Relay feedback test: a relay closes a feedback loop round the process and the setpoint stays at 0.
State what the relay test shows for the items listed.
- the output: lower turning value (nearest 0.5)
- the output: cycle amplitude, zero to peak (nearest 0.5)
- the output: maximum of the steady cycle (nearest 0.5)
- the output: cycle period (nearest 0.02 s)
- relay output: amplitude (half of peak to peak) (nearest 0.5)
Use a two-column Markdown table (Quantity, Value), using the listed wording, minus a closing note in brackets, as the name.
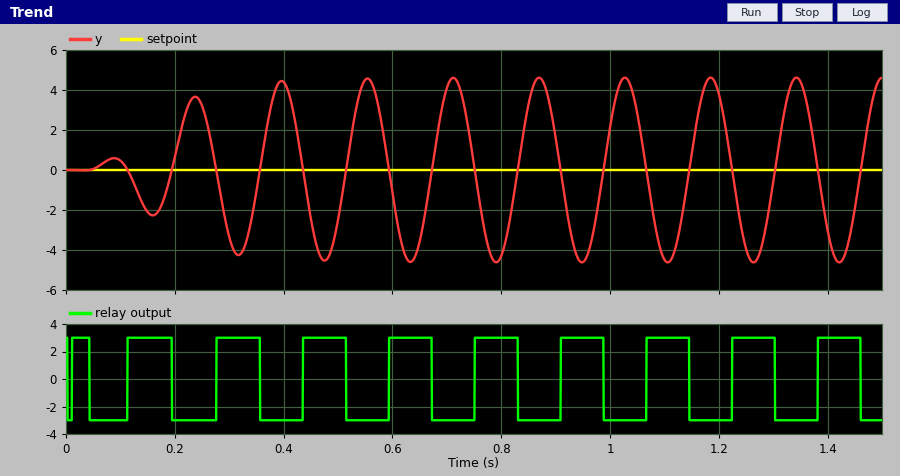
| Quantity | Value |
|---|---|
| the output: lower turning value | -4.5 |
| the output: cycle amplitude, zero to peak | 4.5 |
| the output: maximum of the steady cycle | 4.5 |
| the output: cycle period | 0.16 s |
| relay output: amplitude (half of peak to peak) | 3.0 |
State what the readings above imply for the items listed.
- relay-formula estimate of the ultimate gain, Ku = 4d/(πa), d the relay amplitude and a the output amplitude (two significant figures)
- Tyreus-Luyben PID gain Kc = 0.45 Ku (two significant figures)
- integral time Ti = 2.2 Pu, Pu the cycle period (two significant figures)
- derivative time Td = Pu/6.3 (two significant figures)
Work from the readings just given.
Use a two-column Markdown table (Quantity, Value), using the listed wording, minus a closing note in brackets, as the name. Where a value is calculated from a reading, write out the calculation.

| Quantity | Value |
|---|---|
| relay-formula estimate of the ultimate gain, Ku = 4d/(πa), d the relay amplitude and a the output amplitude | 4 × 3 / (π × 4.5) = 0.85 |
| Tyreus-Luyben PID gain Kc = 0.45 Ku | 0.45 × 0.85 = 0.38 |
| integral time Ti = 2.2 Pu, Pu the cycle period | 2.2 × 0.16 = 0.35 s |
| derivative time Td = Pu/6.3 | 0.16 / 6.3 = 0.025 s |
